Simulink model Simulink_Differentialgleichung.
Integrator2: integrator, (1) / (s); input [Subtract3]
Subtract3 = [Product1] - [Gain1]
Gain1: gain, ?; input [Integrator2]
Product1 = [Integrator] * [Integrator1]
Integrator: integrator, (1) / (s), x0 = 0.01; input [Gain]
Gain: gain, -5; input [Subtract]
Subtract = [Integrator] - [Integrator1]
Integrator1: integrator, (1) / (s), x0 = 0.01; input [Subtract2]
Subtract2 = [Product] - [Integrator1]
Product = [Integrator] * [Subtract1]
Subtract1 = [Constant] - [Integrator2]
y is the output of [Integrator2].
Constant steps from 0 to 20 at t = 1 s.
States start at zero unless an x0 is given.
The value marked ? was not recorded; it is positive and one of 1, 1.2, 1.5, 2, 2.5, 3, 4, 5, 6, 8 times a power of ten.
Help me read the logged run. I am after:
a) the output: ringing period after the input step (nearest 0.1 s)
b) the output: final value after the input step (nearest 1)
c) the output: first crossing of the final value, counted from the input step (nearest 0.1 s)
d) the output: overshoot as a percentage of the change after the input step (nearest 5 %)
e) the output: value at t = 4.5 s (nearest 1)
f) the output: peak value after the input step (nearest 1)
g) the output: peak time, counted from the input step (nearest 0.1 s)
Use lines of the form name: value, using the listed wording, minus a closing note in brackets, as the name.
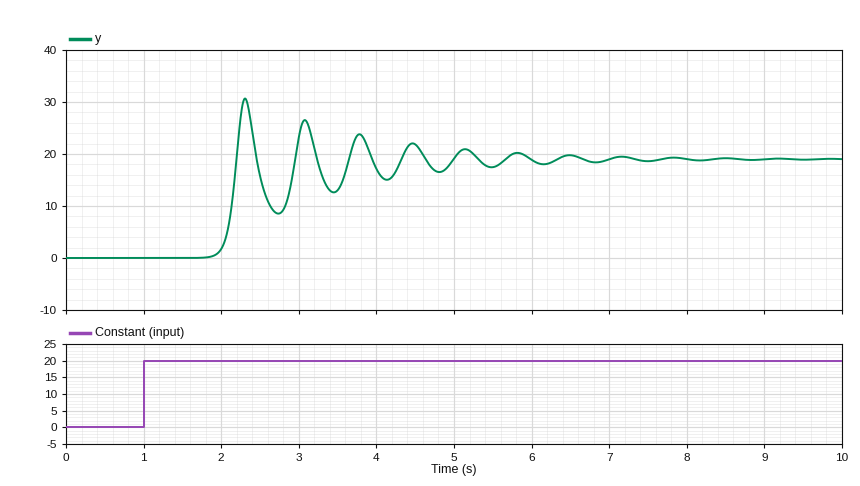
the output: ringing period after the input step: 0.8 s
the output: final value after the input step: 19
the output: first crossing of the final value, counted from the input step: 1.2 s
the output: overshoot as a percentage of the change after the input step: 60 %
the output: value at t = 4.5 s: 22
the output: peak value after the input step: 31
the output: peak time, counted from the input step: 1.3 s
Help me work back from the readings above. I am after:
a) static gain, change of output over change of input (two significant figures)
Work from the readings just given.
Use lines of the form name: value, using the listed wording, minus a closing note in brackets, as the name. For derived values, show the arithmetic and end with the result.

static gain, change of output over change of input: (19 - 0) / (20 - 0) = 0.95
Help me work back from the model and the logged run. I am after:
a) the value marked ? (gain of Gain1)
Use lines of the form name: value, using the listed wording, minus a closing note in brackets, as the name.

the value marked ?: 4
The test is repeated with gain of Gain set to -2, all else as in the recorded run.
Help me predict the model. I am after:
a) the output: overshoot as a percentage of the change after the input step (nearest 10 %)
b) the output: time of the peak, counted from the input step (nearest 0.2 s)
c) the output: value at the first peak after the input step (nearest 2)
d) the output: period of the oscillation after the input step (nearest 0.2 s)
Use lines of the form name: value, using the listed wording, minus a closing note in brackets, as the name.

the output: overshoot as a percentage of the change after the input step: 50 %
the output: time of the peak, counted from the input step: 1.8 s
the output: value at the first peak after the input step: 28
the output: period of the oscillation after the input step: 0.8 s
